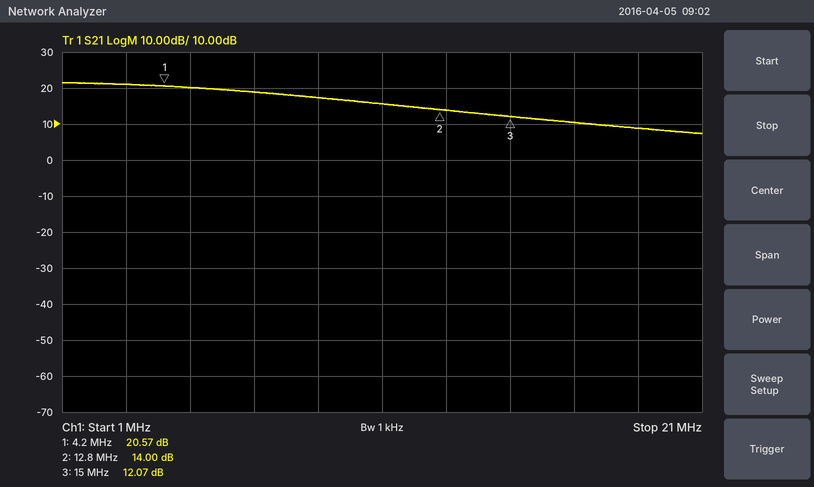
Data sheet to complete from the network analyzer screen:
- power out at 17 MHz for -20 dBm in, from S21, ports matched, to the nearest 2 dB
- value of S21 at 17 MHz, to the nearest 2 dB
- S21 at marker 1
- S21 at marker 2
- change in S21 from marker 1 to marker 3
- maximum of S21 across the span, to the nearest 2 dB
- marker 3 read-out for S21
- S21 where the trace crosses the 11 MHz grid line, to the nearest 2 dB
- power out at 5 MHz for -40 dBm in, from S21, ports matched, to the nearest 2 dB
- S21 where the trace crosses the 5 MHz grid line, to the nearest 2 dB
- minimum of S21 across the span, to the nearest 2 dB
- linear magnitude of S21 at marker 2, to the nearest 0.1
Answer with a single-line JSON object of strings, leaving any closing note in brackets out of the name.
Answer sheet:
{"power out at 17 MHz for -20 dBm in, from S21, ports matched, to the nearest 2 dB": "-10 dBm", "value of S21 at 17 MHz, to the nearest 2 dB": "10 dB", "S21 at marker 1": "20.57 dB", "S21 at marker 2": "14.00 dB", "change in S21 from marker 1 to marker 3": "-8.50 dB", "maximum of S21 across the span, to the nearest 2 dB": "22 dB", "marker 3 read-out for S21": "12.07 dB", "S21 where the trace crosses the 11 MHz grid line, to the nearest 2 dB": "16 dB", "power out at 5 MHz for -40 dBm in, from S21, ports matched, to the nearest 2 dB": "-20 dBm", "S21 where the trace crosses the 5 MHz grid line, to the nearest 2 dB": "20 dB", "minimum of S21 across the span, to the nearest 2 dB": "8 dB", "linear magnitude of S21 at marker 2, to the nearest 0.1": "5.0"}
